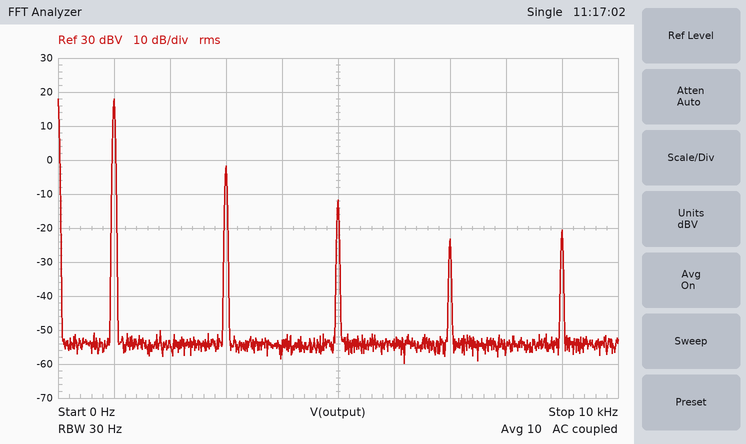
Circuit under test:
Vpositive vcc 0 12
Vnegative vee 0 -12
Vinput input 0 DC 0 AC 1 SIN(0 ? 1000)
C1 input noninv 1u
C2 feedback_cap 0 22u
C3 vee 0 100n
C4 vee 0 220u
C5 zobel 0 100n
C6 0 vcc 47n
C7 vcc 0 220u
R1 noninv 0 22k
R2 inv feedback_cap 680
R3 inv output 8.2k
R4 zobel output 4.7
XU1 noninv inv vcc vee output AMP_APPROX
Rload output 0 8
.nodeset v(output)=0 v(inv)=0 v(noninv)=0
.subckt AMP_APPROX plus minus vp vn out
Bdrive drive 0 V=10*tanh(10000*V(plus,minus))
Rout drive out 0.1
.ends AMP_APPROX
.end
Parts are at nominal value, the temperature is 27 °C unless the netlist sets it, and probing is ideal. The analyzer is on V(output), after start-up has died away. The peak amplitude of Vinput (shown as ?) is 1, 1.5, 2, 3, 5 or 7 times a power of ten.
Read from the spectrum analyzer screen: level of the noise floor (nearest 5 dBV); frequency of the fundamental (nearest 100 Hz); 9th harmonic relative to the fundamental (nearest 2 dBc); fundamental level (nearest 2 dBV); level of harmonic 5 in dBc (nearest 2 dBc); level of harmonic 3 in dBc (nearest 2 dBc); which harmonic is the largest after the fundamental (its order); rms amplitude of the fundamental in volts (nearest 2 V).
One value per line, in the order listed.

-55 dBV
1.0 kHz
-38 dBc
18 dBV
-30 dBc
-20 dBc
3
8 V
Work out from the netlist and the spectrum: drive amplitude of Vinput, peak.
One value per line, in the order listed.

1 V
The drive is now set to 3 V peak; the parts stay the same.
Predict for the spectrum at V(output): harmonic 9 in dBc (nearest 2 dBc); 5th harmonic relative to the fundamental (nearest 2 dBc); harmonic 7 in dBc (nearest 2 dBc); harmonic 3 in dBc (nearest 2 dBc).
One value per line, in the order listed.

-28 dBc
-16 dBc
-22 dBc
-10 dBc
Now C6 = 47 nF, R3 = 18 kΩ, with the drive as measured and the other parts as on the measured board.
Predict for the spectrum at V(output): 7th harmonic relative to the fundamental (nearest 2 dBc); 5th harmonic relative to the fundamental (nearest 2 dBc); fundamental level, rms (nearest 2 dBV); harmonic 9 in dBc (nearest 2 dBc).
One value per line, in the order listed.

-30 dBc
-20 dBc
18 dBV
-48 dBc
